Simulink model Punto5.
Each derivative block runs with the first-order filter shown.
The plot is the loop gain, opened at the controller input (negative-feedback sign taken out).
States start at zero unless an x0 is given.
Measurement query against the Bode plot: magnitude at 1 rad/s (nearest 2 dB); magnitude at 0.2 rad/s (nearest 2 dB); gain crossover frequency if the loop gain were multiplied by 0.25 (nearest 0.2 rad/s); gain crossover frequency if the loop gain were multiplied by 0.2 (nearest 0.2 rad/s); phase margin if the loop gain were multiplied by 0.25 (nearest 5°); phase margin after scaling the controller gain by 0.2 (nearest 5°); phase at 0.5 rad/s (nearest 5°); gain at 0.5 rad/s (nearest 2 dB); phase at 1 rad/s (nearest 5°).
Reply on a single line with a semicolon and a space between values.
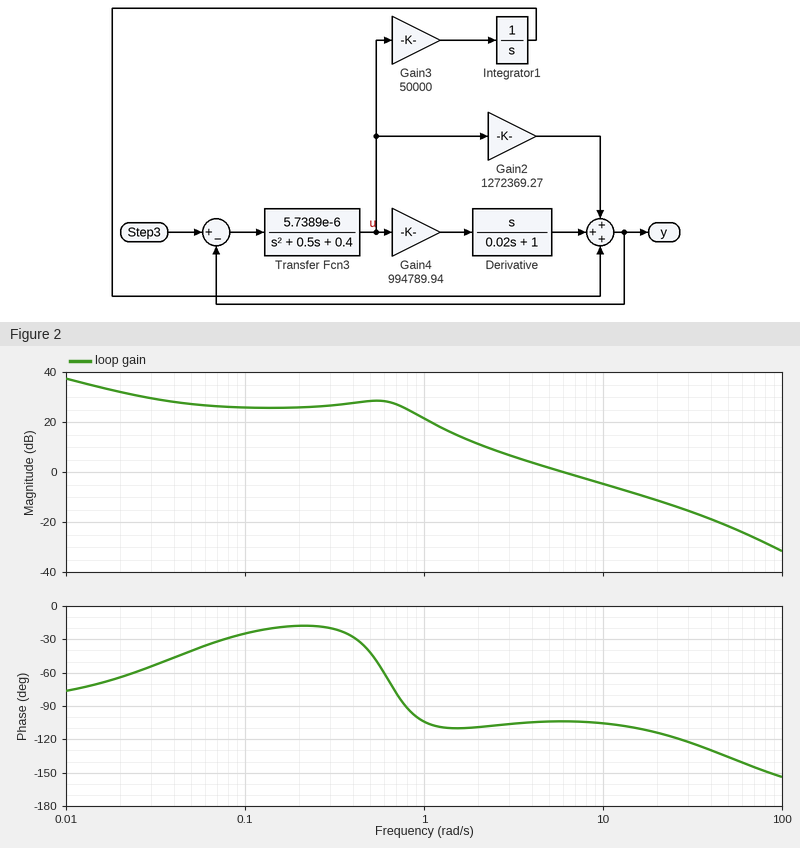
22 dB; 26 dB; 1.8 rad/s; 1.6 rad/s; 70°; 70°; -40°; 28 dB; -105°
